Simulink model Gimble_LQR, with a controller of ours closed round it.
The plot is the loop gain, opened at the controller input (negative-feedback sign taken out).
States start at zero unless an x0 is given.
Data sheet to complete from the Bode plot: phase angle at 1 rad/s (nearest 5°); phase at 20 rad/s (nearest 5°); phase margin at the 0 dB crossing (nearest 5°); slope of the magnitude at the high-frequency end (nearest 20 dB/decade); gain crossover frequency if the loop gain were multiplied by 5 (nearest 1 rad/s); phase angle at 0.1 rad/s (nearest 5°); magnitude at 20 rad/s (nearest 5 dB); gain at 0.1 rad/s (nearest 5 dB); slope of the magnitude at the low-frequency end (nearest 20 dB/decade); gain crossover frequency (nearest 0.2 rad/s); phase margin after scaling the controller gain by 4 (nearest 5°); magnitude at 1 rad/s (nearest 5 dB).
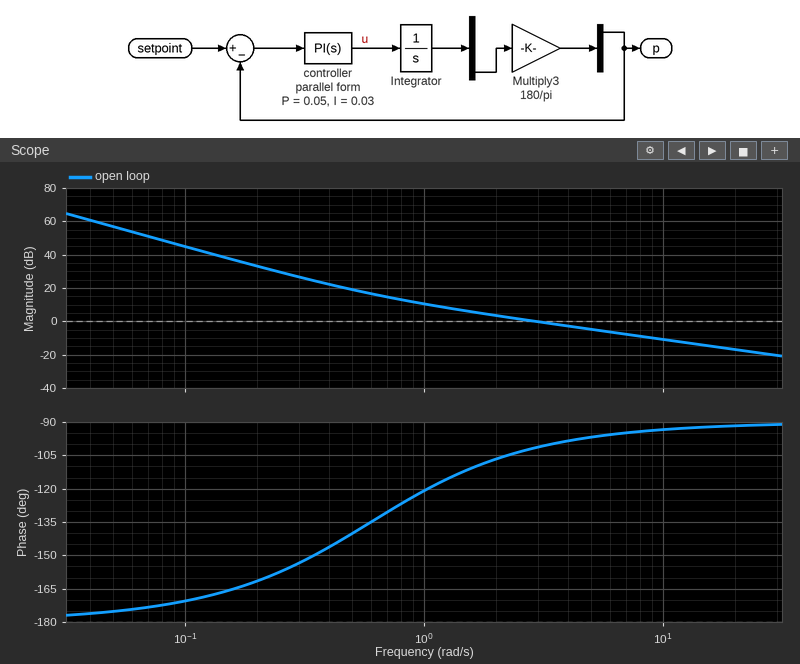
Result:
-120°
-90°
80°
-20 dB/decade
14 rad/s
-170°
-15 dB
45 dB
-40 dB/decade
3.0 rad/s
85°
10 dB
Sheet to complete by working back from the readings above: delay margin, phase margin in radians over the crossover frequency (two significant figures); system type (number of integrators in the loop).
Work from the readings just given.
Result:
0.47 s
2
